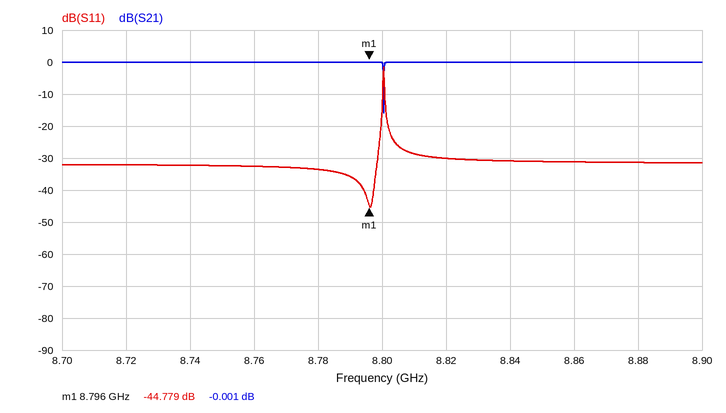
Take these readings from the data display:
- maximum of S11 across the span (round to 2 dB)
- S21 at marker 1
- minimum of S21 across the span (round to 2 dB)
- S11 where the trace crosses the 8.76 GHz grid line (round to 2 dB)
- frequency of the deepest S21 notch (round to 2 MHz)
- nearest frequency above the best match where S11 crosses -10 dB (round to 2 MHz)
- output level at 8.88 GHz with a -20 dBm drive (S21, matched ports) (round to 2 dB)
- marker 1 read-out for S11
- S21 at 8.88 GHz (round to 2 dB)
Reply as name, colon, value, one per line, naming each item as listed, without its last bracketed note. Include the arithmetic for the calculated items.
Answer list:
maximum of S11 across the span: -2 dB
S21 at marker 1: -0.001 dB
minimum of S21 across the span: -16 dB
S11 where the trace crosses the 8.76 GHz grid line: -32 dB
frequency of the deepest S21 notch: 8.800 GHz
nearest frequency above the best match where S11 crosses -10 dB: 8.800 GHz
output level at 8.88 GHz with a -20 dBm drive (S21, matched ports): -20 dBm + (0 dB) = -20 dBm
marker 1 read-out for S11: -44.779 dB
S21 at 8.88 GHz: 0 dB
